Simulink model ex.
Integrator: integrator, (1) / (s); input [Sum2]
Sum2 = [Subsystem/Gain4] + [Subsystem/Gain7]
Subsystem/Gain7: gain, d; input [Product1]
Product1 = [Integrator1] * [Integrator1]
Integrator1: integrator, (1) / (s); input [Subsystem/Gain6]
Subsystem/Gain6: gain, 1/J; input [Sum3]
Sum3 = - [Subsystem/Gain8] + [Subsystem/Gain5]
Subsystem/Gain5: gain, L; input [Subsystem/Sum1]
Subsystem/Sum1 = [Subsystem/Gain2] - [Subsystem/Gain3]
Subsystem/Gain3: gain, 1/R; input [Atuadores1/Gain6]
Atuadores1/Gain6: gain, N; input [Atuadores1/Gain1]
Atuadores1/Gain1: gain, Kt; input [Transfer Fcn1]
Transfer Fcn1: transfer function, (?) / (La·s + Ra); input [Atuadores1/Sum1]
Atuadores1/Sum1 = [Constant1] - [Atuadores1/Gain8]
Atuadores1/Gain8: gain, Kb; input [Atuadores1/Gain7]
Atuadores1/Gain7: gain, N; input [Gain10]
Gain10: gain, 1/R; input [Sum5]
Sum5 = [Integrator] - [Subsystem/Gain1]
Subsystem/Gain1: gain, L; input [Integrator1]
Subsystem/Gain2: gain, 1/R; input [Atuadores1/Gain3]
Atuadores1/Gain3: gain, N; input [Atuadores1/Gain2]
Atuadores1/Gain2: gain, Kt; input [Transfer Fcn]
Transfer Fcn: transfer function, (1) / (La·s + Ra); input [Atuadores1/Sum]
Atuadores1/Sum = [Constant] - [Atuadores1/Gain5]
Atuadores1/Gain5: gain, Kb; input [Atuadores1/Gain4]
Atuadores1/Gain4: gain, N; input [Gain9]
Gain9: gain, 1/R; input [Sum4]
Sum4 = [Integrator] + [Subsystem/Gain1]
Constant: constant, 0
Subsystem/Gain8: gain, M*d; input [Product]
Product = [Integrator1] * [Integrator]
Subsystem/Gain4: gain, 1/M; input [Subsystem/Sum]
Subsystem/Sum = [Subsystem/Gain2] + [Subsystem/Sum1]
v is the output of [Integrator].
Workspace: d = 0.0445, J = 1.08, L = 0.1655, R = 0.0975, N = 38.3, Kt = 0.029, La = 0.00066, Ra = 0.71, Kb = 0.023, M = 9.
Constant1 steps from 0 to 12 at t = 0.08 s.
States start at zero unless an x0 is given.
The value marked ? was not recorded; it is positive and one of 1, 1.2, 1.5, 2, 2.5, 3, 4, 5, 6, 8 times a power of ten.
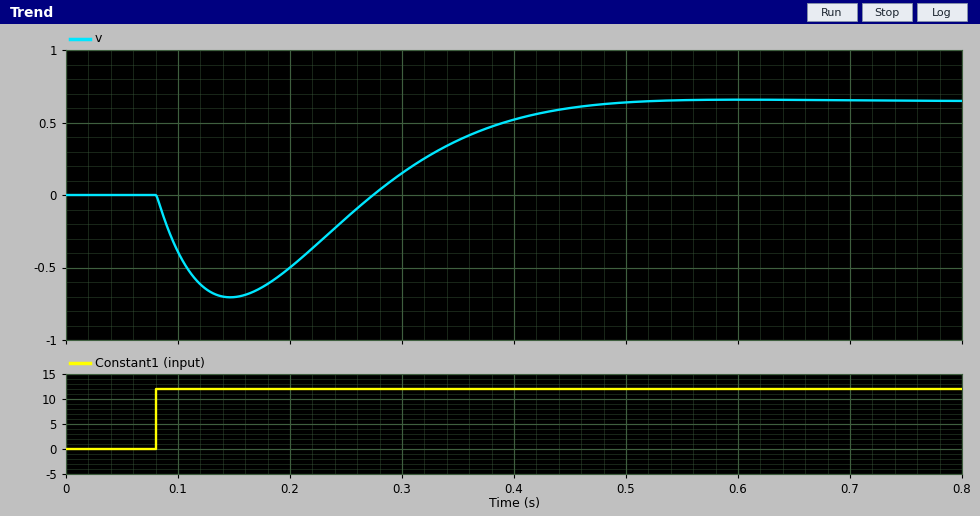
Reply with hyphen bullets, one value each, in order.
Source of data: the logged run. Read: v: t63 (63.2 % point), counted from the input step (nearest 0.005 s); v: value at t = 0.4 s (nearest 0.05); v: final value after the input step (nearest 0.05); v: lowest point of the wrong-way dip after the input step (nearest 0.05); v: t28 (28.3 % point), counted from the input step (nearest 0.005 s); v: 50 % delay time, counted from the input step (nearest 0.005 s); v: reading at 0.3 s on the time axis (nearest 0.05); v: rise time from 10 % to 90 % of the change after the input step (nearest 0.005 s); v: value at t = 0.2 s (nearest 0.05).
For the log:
- 0.280 s
- 0.50
- 0.65
- -0.70
- 0.225 s
- 0.255 s
- 0.15
- 0.150 s
- -0.50
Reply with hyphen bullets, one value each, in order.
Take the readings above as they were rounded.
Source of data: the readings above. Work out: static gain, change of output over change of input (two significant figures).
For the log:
- 0.054
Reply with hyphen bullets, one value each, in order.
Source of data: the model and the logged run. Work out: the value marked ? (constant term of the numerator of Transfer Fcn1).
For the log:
- 1.2
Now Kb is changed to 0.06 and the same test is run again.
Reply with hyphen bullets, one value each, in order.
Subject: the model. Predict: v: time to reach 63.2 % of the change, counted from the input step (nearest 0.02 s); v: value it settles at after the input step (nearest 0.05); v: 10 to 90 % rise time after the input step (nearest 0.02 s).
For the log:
- 0.12 s
- 0.25
- 0.06 s
